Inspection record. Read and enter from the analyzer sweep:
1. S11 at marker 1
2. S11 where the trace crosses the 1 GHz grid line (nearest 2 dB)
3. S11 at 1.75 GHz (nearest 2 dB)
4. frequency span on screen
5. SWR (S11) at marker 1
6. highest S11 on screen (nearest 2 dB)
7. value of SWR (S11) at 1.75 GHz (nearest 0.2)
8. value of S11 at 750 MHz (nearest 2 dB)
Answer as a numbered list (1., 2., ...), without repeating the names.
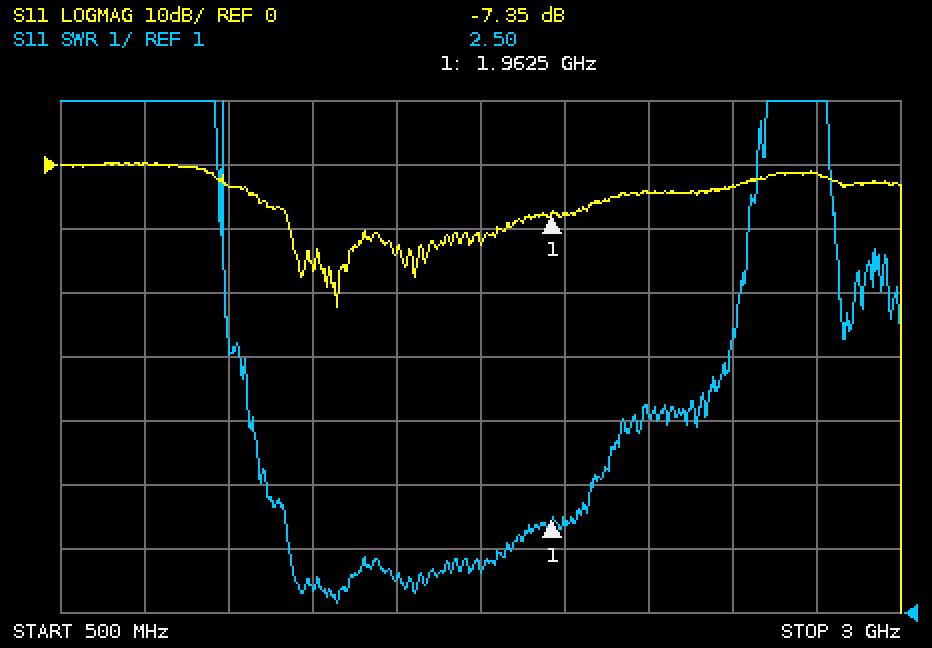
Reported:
1. -7.35 dB
2. -4 dB
3. -12 dB
4. 2.5 GHz
5. 2.50
6. 0 dB
7. 1.6
8. 0 dB
